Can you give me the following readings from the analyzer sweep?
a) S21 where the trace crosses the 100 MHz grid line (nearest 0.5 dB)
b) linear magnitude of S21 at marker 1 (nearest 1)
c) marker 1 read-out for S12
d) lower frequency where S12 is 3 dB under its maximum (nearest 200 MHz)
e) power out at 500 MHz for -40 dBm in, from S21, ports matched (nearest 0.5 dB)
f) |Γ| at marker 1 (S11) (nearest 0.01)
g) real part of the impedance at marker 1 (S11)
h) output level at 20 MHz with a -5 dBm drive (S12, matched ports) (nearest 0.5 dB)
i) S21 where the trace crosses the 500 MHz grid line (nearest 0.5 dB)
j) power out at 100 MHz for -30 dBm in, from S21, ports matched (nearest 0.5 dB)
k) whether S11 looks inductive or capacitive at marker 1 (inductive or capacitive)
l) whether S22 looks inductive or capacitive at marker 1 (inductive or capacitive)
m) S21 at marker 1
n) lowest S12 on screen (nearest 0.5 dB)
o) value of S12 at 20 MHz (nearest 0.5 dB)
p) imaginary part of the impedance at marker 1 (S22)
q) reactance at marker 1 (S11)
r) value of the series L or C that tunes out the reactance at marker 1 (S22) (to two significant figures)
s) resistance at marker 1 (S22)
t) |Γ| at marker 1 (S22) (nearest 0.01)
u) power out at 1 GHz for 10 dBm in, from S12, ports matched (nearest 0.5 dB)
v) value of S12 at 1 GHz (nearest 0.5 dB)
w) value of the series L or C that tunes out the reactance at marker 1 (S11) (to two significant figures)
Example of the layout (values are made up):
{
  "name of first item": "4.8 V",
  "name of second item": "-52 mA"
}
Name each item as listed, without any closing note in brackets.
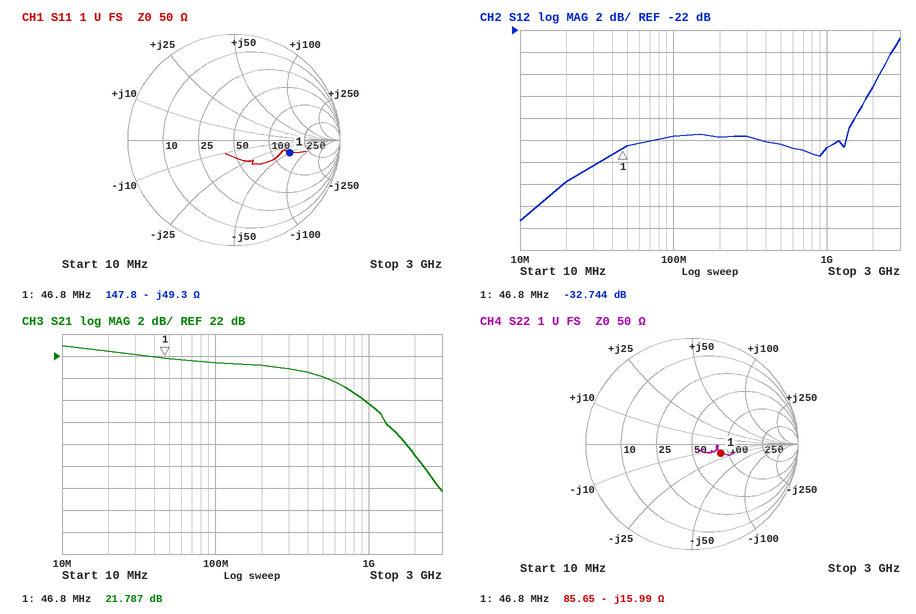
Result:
{
  "S21 where the trace crosses the 100 MHz grid line": "21.5 dB",
  "linear magnitude of S21 at marker 1": "12",
  "marker 1 read-out for S12": "-32.744 dB",
  "lower frequency where S12 is 3 dB under its maximum": "2.2 GHz",
  "power out at 500 MHz for -40 dBm in, from S21, ports matched": "-20.0 dBm",
  "|Γ| at marker 1 (S11)": "0.54",
  "real part of the impedance at marker 1": "147.8 Ω",
  "output level at 20 MHz with a -5 dBm drive (S12, matched ports)": "-41.0 dBm",
  "S21 where the trace crosses the 500 MHz grid line": "20.0 dB",
  "power out at 100 MHz for -30 dBm in, from S21, ports matched": "-8.5 dBm",
  "whether S11 looks inductive or capacitive at marker 1": "capacitive",
  "whether S22 looks inductive or capacitive at marker 1": "capacitive",
  "S21 at marker 1": "21.787 dB",
  "lowest S12 on screen": "-39.5 dB",
  "value of S12 at 20 MHz": "-36.0 dB",
  "imaginary part of the impedance at marker 1": "-15.99 Ω",
  "reactance at marker 1": "-49.3 Ω",
  "value of the series L or C that tunes out the reactance at marker 1 (S22)": "54 nH",
  "resistance at marker 1": "85.65 Ω",
  "|Γ| at marker 1 (S22)": "0.29",
  "power out at 1 GHz for 10 dBm in, from S12, ports matched": "-22.5 dBm",
  "value of S12 at 1 GHz": "-32.5 dB",
  "value of the series L or C that tunes out the reactance at marker 1 (S11)": "170 nH"
}
